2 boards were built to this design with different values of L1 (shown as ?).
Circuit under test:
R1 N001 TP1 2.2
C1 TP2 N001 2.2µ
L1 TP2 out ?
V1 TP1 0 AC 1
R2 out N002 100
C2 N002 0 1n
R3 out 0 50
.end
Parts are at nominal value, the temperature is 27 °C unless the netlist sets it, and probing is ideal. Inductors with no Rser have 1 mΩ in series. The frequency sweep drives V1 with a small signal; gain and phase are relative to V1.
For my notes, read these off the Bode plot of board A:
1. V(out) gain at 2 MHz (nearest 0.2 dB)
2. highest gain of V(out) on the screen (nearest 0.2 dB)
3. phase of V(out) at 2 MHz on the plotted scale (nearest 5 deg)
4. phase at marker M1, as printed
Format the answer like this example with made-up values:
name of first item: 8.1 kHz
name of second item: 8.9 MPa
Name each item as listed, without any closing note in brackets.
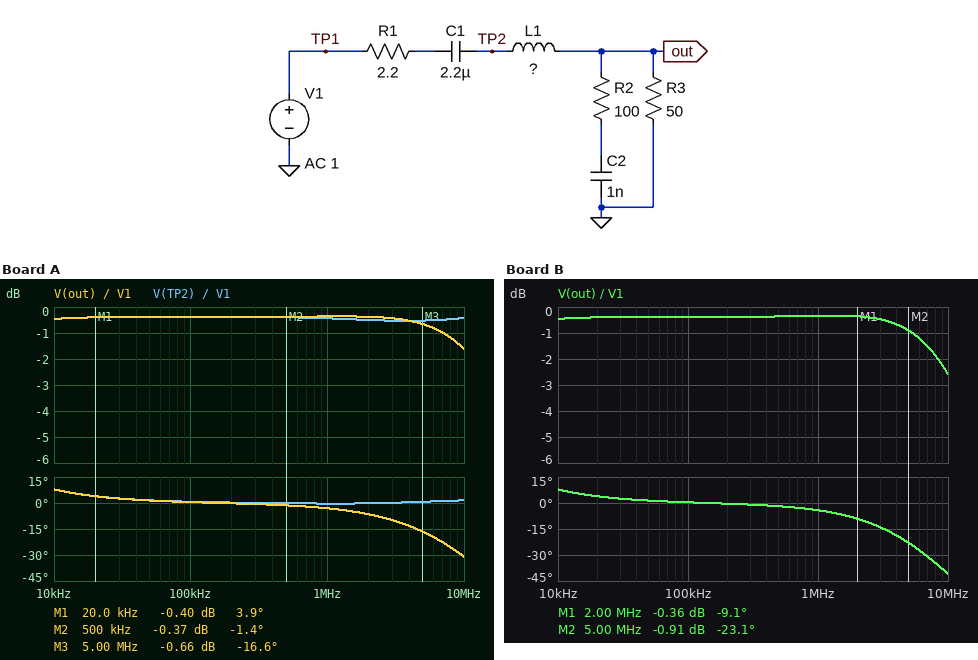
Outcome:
V(out) gain at 2 MHz: -0.4 dB
highest gain of V(out) on the screen: -0.4 dB
phase of V(out) at 2 MHz on the plotted scale: -5 deg
phase at marker M1, as printed: 3.9 deg
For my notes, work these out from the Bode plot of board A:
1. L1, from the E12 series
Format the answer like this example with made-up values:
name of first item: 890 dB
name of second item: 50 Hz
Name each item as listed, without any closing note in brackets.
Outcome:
L1, from the E12 series: 330 nH
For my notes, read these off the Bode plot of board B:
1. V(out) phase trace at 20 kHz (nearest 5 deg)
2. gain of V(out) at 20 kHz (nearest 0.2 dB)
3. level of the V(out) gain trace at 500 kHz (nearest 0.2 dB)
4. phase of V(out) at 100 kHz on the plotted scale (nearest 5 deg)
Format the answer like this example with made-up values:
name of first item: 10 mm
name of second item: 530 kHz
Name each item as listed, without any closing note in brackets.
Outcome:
V(out) phase trace at 20 kHz: 5 deg
gain of V(out) at 20 kHz: -0.4 dB
level of the V(out) gain trace at 500 kHz: -0.4 dB
phase of V(out) at 100 kHz on the plotted scale: 0 deg
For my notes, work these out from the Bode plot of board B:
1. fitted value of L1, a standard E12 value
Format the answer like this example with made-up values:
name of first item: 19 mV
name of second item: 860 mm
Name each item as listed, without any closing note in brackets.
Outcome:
fitted value of L1, a standard E12 value: 470 nH
